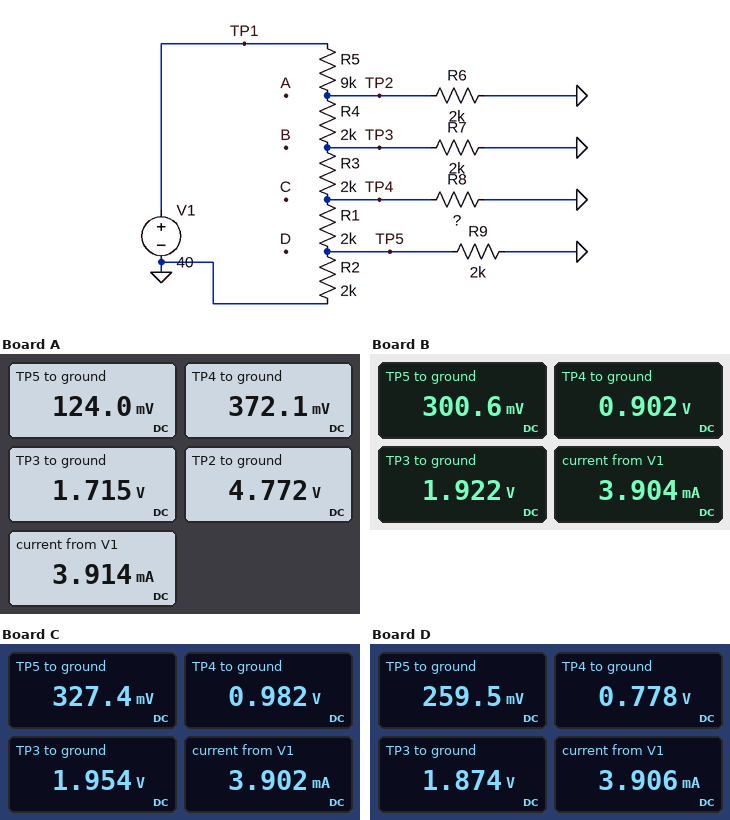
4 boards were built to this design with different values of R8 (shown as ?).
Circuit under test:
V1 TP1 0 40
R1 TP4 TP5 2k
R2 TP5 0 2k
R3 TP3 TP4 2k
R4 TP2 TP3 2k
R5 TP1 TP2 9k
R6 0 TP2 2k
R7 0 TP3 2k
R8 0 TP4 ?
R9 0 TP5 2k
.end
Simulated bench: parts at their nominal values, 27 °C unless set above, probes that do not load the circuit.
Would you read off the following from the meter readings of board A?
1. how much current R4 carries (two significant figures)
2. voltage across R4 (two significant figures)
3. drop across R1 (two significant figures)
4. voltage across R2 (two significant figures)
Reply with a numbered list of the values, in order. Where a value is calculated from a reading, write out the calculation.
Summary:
1. (4.772 V - 1.715 V) / 2 kΩ = 1.5 mA
2. 4.772 V - 1.715 V = 3.1 V
3. 372.1 mV - 124 mV = 250 mV
4. 124 mV = 120 mV
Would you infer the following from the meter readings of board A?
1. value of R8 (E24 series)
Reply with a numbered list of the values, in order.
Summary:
1. 680 Ω
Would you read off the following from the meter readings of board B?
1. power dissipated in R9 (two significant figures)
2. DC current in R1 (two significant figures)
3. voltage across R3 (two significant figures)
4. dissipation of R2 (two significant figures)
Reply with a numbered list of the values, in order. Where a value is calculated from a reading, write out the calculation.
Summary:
1. (300.6 mV)^2 / 2 kΩ = 45 µW
2. (902 mV - 300.6 mV) / 2 kΩ = 300 µA
3. 1.922 V - 902 mV = 1.0 V
4. (300.6 mV)^2 / 2 kΩ = 45 µW
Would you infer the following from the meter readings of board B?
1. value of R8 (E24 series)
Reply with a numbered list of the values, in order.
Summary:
1. 4.3 kΩ
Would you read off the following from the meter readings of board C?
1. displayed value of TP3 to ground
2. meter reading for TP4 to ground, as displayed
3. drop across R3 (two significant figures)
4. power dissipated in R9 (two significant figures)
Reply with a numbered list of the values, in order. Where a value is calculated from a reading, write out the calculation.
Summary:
1. 1.954 V
2. 0.982 V
3. 1.954 V - 982 mV = 970 mV
4. (327.4 mV)^2 / 2 kΩ = 54 µW
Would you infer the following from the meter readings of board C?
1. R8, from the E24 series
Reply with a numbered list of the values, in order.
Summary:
1. 6.2 kΩ
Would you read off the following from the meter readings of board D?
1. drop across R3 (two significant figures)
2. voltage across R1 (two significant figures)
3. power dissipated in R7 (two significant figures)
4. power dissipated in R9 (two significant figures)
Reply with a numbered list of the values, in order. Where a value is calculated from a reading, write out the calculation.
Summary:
1. 1.874 V - 778 mV = 1.1 V
2. 778 mV - 259.5 mV = 520 mV
3. (1.874 V)^2 / 2 kΩ = 1.8 mW
4. (259.5 mV)^2 / 2 kΩ = 34 µW
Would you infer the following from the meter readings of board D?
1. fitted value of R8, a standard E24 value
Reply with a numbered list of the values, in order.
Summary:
1. 2.7 kΩ
